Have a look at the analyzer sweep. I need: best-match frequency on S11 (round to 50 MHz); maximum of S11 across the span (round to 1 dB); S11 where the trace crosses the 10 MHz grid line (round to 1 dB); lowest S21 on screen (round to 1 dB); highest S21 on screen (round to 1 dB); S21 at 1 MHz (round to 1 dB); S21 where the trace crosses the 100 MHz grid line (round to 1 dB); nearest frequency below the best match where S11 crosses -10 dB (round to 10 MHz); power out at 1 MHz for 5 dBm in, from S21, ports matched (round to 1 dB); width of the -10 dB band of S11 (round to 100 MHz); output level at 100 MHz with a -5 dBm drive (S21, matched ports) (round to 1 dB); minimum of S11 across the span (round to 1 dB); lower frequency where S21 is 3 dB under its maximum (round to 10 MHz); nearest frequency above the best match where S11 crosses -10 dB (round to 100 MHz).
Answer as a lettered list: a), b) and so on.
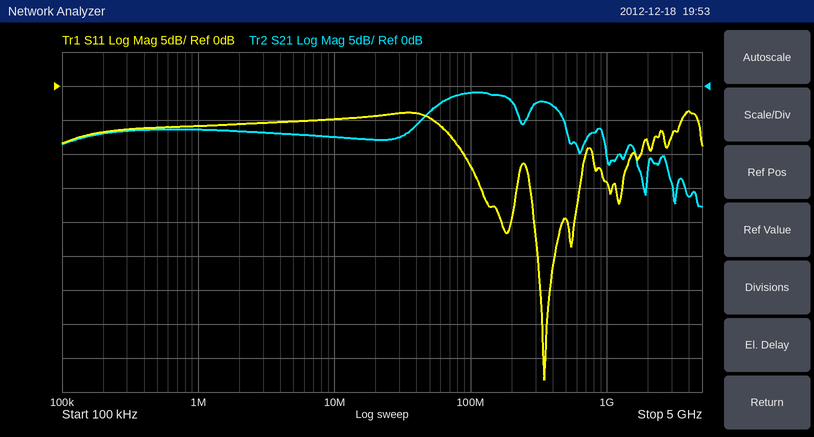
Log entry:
a) 350 MHz
b) -4 dB
c) -5 dB
d) -18 dB
e) -1 dB
f) -6 dB
g) -1 dB
h) 90 MHz
i) -1 dBm
j) 600 MHz
k) -6 dBm
l) -43 dB
m) 50 MHz
n) 700 MHz
